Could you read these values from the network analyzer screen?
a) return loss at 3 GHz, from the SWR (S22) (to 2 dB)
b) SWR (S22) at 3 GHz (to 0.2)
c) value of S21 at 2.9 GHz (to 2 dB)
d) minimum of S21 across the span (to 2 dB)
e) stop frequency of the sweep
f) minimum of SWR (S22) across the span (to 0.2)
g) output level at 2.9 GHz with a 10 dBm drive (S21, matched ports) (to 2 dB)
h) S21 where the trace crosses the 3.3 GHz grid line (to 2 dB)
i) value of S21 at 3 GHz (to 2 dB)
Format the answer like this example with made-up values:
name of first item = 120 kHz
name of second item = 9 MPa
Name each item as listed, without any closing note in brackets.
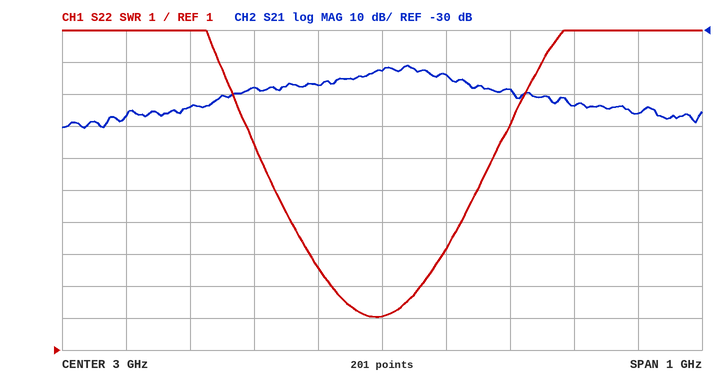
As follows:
return loss at 3 GHz, from the SWR (S22) = 10 dB
SWR (S22) at 3 GHz = 2.0
value of S21 at 2.9 GHz = -48 dB
minimum of S21 across the span = -60 dB
stop frequency of the sweep = 3.5 GHz
minimum of SWR (S22) across the span = 2.0
output level at 2.9 GHz with a 10 dBm drive (S21, matched ports) = -38 dBm
S21 where the trace crosses the 3.3 GHz grid line = -54 dB
value of S21 at 3 GHz = -42 dB
